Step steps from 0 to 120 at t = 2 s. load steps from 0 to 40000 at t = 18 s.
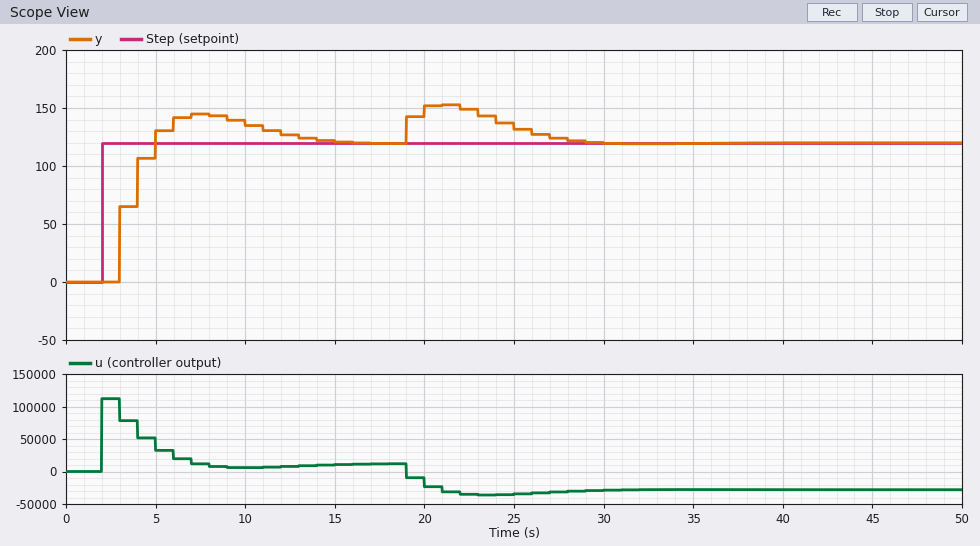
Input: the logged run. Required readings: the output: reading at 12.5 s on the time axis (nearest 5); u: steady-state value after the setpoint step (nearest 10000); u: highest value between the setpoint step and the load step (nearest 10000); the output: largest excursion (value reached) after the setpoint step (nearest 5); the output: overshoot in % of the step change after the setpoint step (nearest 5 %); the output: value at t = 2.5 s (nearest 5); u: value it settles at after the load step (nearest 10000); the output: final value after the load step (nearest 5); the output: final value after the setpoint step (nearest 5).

125
10000
110000
145
20 %
0
-30000
120
120
